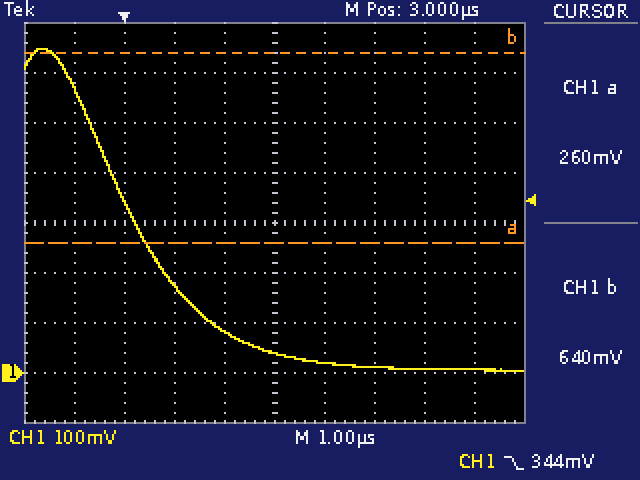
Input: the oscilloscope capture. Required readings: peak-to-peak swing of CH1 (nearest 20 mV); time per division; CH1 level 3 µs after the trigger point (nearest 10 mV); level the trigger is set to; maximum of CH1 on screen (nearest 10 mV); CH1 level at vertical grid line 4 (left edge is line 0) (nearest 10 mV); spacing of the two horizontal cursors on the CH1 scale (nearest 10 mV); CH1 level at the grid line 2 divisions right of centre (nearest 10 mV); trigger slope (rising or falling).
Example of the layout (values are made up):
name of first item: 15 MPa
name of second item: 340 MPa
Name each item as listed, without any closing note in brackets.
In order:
peak-to-peak swing of CH1: 640 mV
time per division: 1 µs
CH1 level 3 µs after the trigger point: 40 mV
level the trigger is set to: 344 mV
maximum of CH1 on screen: 650 mV
CH1 level at vertical grid line 4 (left edge is line 0): 80 mV
spacing of the two horizontal cursors on the CH1 scale: 380 mV
CH1 level at the grid line 2 divisions right of centre: 10 mV
trigger slope: falling
